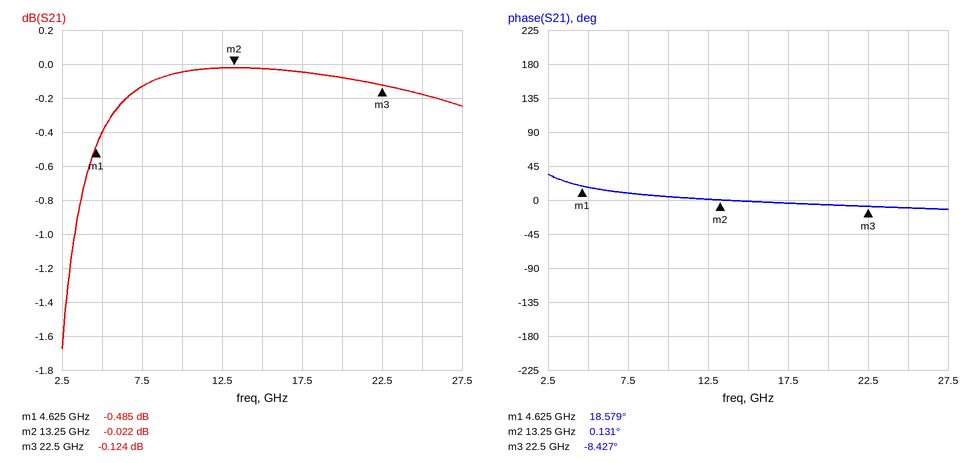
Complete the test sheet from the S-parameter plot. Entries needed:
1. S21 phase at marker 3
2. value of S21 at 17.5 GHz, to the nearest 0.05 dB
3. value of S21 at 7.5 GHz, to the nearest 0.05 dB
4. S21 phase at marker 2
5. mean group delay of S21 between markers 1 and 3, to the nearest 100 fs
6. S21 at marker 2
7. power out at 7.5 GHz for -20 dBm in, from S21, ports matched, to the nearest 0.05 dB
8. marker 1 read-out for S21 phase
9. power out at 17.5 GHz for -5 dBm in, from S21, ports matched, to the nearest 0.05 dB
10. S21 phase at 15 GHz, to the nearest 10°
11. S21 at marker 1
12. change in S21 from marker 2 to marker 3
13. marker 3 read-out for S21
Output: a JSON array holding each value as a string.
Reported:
["-8.427°", "-0.05 dB", "-0.15 dB", "0.131°", "4.2 ps", "-0.022 dB", "-20.15 dBm", "18.579°", "-5.05 dBm", "0°", "-0.485 dB", "-0.102 dB", "-0.124 dB"]
